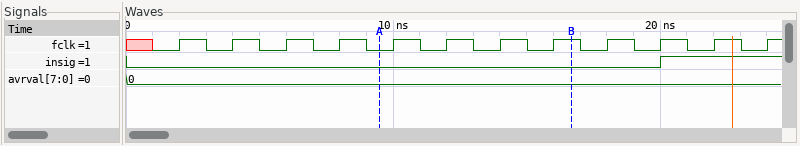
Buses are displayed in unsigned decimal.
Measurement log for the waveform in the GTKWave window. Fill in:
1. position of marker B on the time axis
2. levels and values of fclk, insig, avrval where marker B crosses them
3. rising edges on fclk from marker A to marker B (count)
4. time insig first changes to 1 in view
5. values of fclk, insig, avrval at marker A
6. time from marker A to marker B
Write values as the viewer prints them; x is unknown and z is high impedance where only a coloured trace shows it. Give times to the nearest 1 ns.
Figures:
17 ns
fclk=1, insig=0, avrval=0
4
20 ns
fclk=0, insig=0, avrval=0
7 ns
